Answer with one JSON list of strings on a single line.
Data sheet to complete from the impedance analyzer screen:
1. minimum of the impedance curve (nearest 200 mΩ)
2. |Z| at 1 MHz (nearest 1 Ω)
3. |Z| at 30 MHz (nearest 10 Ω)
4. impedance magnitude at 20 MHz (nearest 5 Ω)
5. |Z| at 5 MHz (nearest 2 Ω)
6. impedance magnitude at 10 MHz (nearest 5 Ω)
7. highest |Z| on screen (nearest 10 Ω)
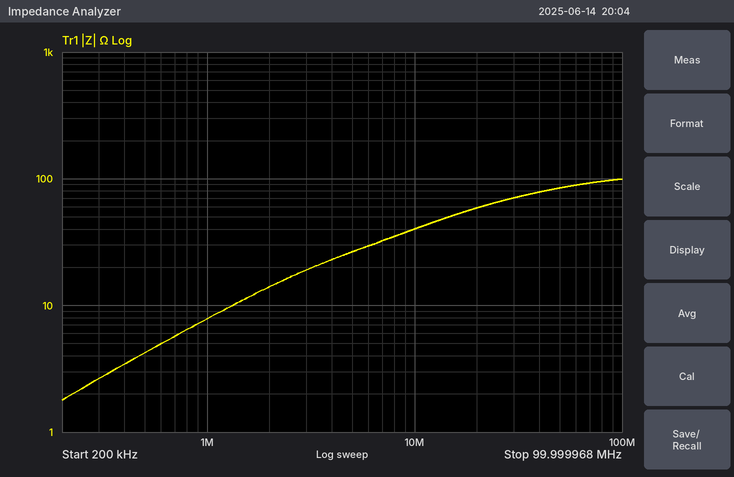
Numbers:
["1.8 Ω", "8 Ω", "70 Ω", "60 Ω", "26 Ω", "40 Ω", "100 Ω"]
